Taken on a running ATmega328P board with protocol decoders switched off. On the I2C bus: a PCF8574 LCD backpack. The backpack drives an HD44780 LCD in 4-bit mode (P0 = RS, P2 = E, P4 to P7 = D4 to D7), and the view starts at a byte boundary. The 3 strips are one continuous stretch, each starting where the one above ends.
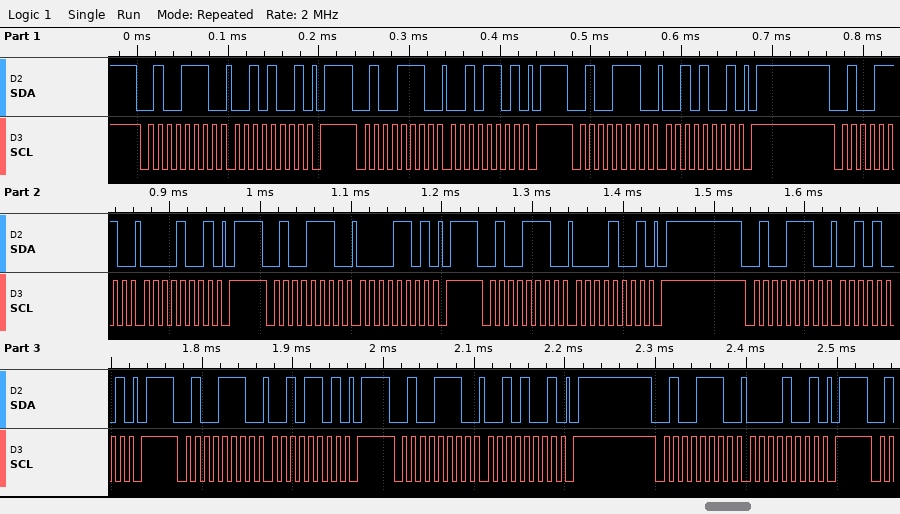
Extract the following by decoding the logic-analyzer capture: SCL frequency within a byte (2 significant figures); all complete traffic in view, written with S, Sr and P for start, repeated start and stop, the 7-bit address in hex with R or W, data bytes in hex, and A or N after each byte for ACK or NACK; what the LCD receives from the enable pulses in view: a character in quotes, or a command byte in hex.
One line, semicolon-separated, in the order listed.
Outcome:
100 kHz; S 27W A 29 A P S 27W A 2D A P S 27W A 29 A P S 27W A 09 A P S 27W A 0D A P S 27W A 09 A P S 27W A 29 A P S 27W A 2D A P S 27W A 29 A P S 27W A 09 A P; ' '
